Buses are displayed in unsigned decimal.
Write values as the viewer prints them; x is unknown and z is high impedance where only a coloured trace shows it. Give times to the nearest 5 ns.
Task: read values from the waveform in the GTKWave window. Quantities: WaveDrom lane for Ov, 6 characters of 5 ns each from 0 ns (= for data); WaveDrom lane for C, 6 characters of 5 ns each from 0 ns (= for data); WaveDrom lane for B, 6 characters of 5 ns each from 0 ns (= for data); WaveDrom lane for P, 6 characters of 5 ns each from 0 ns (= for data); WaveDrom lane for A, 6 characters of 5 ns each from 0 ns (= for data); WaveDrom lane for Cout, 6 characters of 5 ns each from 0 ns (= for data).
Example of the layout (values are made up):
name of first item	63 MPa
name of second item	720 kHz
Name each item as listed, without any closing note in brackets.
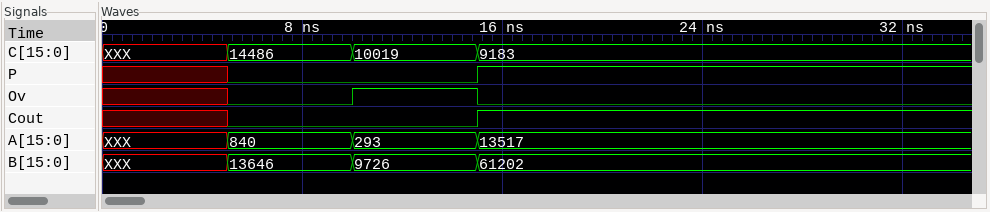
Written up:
WaveDrom lane for Ov, 6 characters of 5 ns each from 0 ns	{name: 'Ov', wave: 'x010..'}
WaveDrom lane for C, 6 characters of 5 ns each from 0 ns	{name: 'C', wave: 'x===..', data: '14486 10019 9183'}
WaveDrom lane for B, 6 characters of 5 ns each from 0 ns	{name: 'B', wave: 'x===..', data: '13646 9726 61202'}
WaveDrom lane for P, 6 characters of 5 ns each from 0 ns	{name: 'P', wave: 'x0.1..'}
WaveDrom lane for A, 6 characters of 5 ns each from 0 ns	{name: 'A', wave: 'x===..', data: '840 293 13517'}
WaveDrom lane for Cout, 6 characters of 5 ns each from 0 ns	{name: 'Cout', wave: 'x0.1..'}
